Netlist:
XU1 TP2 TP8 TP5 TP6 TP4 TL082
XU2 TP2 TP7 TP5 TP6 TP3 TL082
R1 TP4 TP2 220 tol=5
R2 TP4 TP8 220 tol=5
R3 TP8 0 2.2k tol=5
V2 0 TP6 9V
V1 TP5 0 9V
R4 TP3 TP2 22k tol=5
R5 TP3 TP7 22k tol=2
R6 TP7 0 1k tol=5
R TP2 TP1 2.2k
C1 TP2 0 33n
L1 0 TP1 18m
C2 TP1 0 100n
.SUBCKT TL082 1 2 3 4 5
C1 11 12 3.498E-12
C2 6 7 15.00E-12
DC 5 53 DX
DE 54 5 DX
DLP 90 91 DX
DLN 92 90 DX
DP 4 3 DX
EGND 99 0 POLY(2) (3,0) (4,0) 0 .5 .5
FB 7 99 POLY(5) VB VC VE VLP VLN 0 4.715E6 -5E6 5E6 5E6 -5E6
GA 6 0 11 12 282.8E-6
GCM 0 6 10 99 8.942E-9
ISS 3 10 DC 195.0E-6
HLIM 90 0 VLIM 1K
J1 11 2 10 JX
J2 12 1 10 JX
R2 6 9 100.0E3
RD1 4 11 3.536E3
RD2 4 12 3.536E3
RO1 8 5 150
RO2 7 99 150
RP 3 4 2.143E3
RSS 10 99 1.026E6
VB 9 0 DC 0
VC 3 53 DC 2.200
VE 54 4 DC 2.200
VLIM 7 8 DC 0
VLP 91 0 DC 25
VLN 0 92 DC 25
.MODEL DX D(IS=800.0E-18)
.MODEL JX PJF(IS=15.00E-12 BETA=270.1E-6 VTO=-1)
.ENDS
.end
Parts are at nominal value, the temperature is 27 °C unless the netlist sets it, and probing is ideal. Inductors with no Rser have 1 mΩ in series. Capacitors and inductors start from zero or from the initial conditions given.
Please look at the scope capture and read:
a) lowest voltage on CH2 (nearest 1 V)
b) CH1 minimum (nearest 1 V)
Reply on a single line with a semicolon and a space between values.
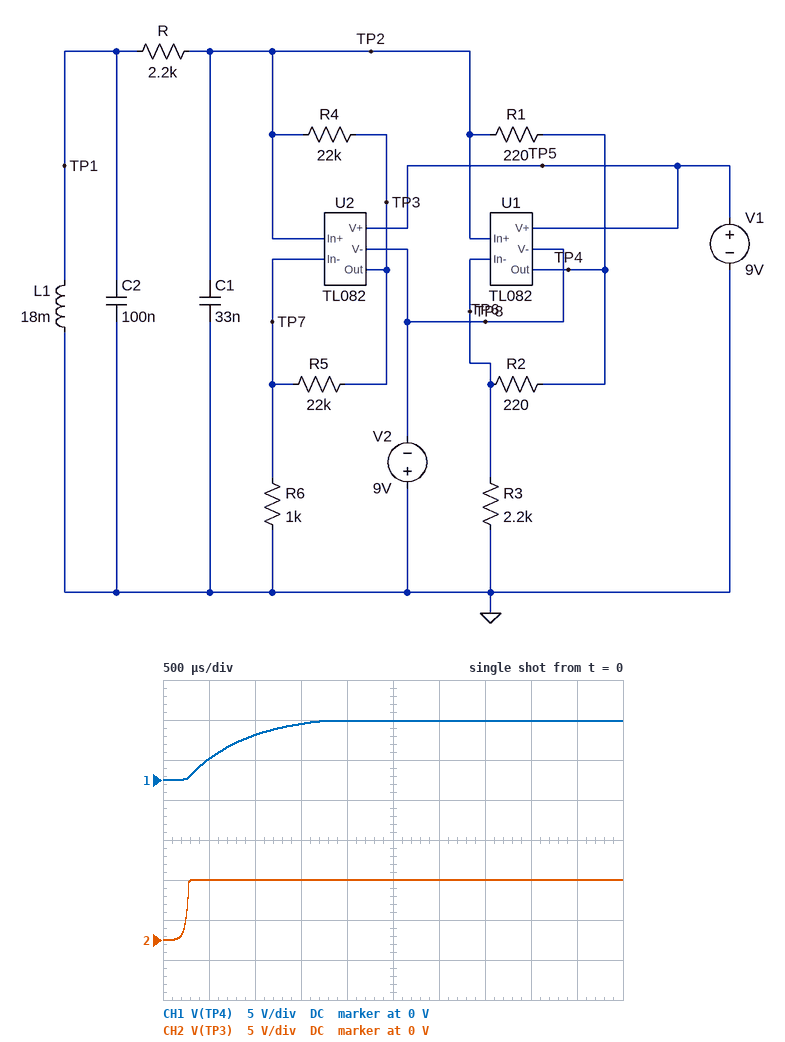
0 V; 0 V
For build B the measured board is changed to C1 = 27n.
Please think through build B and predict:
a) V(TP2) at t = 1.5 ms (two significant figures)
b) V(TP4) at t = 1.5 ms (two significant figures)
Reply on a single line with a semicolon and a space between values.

6.7 V; 7.4 V
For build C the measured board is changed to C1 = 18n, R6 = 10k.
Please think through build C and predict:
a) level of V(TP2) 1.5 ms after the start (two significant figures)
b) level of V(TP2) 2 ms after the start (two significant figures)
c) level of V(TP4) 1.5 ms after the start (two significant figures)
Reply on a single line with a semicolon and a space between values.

5.1 V; 6.7 V; 5.6 V
